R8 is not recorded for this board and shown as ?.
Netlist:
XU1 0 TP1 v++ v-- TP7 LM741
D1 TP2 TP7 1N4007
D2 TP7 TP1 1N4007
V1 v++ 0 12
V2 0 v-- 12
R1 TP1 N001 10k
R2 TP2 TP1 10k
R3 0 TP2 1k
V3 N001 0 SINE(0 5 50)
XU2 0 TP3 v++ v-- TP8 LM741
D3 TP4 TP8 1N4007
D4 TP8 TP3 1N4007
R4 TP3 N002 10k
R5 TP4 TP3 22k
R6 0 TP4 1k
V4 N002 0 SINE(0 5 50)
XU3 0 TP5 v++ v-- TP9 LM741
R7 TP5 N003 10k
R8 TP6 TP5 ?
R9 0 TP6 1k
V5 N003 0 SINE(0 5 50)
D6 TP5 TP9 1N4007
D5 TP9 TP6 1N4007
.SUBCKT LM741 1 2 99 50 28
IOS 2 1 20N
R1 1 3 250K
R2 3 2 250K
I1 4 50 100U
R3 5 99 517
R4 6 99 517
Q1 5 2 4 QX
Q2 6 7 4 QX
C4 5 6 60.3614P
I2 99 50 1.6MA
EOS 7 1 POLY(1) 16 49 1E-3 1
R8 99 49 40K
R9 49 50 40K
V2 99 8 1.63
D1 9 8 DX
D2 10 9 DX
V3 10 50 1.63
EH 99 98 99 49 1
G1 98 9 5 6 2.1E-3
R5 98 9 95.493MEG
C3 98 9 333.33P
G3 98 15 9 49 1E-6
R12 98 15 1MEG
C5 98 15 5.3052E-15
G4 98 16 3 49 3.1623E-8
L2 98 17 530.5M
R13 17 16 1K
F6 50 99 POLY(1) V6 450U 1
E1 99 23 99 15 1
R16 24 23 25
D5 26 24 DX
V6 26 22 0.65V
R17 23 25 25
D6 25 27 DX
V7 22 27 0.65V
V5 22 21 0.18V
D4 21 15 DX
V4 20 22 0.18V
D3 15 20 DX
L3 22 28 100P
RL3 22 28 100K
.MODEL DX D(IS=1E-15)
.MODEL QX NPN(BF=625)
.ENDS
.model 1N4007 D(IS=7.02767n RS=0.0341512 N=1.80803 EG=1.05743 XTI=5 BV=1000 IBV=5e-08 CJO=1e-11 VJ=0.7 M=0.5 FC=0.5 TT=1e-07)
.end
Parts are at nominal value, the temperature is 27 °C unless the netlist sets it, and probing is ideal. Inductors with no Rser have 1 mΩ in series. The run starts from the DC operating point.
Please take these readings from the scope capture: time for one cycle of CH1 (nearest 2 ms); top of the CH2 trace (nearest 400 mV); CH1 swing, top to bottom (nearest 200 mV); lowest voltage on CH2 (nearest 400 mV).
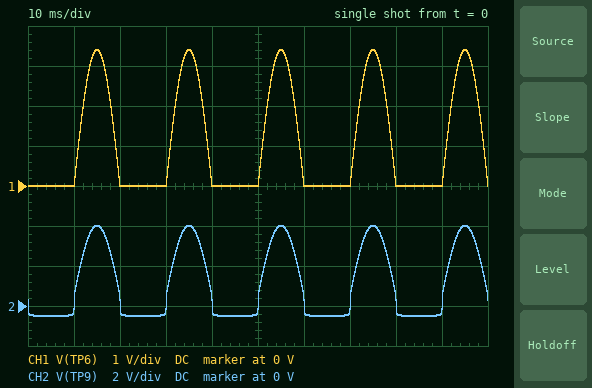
20 ms
4.0 V
3.4 V
-400 mV
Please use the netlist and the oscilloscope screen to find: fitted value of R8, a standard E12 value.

6.8 kΩ
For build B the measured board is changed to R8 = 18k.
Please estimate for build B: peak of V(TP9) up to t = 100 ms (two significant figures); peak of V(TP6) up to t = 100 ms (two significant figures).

9.7 V
9.0 V
